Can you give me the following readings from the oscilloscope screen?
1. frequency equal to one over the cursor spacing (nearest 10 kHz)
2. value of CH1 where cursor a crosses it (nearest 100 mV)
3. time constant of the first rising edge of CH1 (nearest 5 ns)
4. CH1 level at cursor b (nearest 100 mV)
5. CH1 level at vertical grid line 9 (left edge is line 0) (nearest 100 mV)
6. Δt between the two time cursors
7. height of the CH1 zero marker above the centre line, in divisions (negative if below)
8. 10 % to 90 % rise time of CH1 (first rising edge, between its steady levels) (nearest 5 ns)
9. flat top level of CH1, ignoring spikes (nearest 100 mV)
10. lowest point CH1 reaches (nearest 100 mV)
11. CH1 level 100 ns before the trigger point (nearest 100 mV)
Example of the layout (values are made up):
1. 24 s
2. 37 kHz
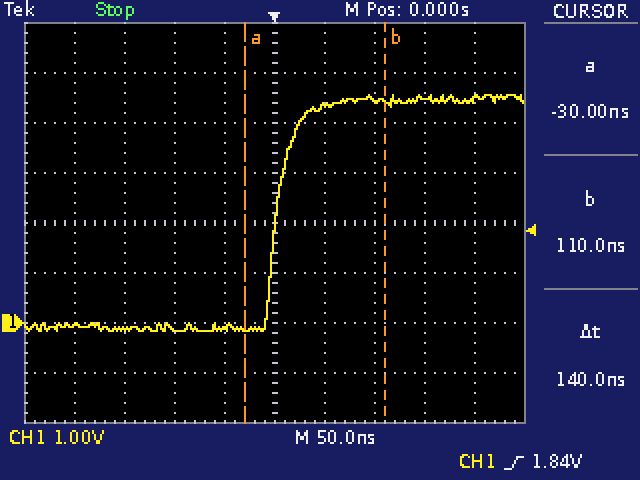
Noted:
1. 7.14 MHz
2. -100 mV
3. 15 ns
4. 4.4 V
5. 4.5 V
6. 140 ns
7. -2.0 div
8. 30 ns
9. 4.5 V
10. -200 mV
11. -100 mV
